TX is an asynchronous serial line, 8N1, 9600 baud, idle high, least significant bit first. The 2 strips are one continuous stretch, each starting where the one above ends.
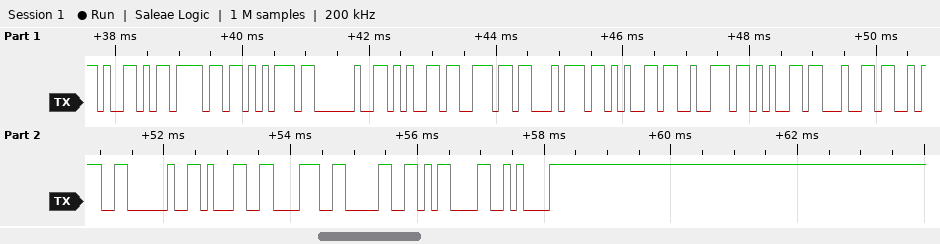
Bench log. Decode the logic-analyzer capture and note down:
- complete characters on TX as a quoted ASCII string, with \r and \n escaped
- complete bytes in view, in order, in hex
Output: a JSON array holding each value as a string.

["\"You entered: 180\\r\\n\"", "0x59 0x6F 0x75 0x20 0x65 0x6E 0x74 0x65 0x72 0x65 0x64 0x3A 0x20 0x31 0x38 0x30 0x0D 0x0A"]
